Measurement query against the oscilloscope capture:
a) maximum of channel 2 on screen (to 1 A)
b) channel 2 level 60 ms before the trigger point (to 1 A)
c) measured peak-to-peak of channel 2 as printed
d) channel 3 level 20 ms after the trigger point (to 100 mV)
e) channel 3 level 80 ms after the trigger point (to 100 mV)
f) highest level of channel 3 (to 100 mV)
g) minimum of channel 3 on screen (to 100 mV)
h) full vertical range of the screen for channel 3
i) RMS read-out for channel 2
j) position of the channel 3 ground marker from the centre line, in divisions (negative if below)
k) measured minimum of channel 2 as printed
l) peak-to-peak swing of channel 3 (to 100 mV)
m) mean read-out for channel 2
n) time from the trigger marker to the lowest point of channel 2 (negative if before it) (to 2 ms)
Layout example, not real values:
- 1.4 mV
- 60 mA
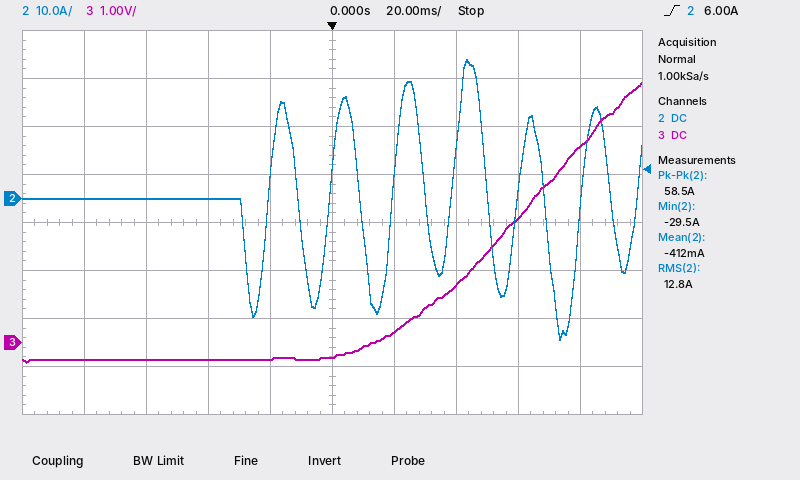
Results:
- 29 A
- 0 A
- 58.5 A
- 200 mV
- 4.1 V
- 5.4 V
- -400 mV
- 8 V
- 12.8 A
- -2.5 div
- -29.5 A
- 5.8 V
- -412 mA
- +74 ms
